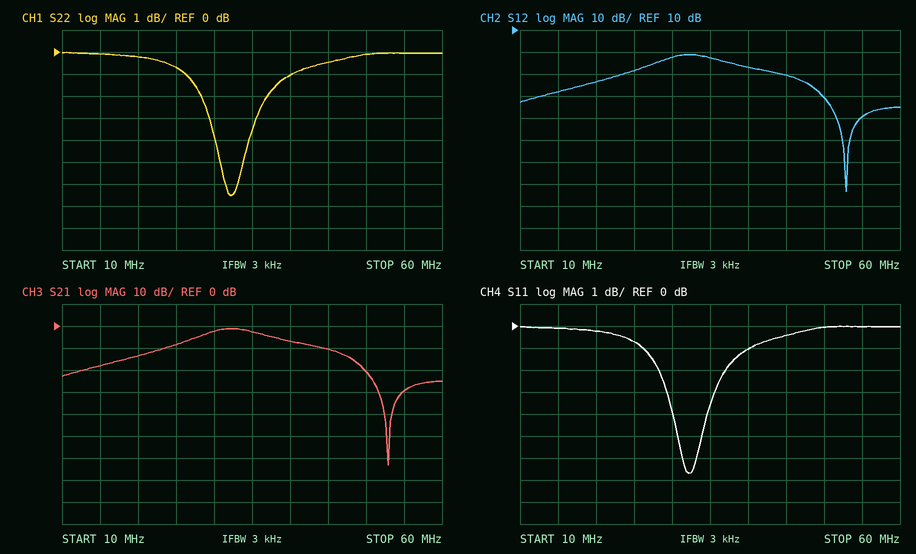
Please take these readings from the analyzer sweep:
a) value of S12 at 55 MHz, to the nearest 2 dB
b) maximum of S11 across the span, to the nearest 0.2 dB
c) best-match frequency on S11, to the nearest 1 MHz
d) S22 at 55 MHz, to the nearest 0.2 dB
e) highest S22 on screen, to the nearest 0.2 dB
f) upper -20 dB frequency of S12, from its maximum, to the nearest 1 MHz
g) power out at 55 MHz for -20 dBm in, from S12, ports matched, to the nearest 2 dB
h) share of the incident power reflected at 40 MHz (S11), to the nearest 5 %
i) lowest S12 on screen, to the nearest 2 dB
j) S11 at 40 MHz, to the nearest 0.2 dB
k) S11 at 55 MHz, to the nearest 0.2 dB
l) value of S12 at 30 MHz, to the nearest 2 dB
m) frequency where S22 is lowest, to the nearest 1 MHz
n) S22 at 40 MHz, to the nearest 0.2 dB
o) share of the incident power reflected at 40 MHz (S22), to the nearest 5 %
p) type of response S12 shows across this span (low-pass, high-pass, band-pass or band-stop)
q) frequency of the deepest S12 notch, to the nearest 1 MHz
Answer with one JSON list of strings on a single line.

["-30 dB", "0.0 dB", "32 MHz", "0.0 dB", "0.0 dB", "50 MHz", "-50 dBm", "80 %", "-64 dB", "-1.0 dB", "0.0 dB", "-2 dB", "32 MHz", "-1.0 dB", "80 %", "band-pass", "53 MHz"]
